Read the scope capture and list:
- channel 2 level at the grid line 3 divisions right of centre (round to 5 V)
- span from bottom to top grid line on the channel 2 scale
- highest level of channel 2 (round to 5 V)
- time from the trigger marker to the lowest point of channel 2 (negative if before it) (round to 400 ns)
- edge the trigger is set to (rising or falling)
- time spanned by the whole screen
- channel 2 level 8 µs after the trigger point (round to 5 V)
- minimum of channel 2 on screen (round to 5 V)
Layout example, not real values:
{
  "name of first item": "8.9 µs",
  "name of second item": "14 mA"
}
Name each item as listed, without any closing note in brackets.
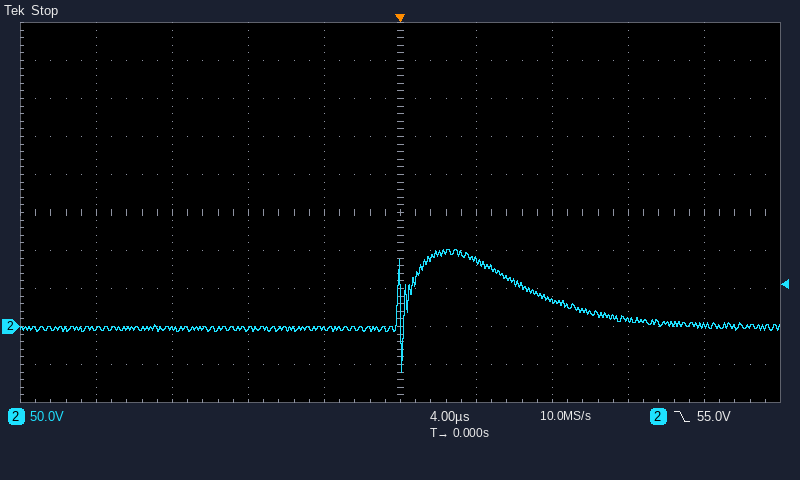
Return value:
{
  "channel 2 level at the grid line 3 divisions right of centre": "10 V",
  "span from bottom to top grid line on the channel 2 scale": "500 V",
  "highest level of channel 2": "100 V",
  "time from the trigger marker to the lowest point of channel 2 (negative if before it)": "0.0 µs",
  "edge the trigger is set to": "falling",
  "time spanned by the whole screen": "40 µs",
  "channel 2 level 8 µs after the trigger point": "35 V",
  "minimum of channel 2 on screen": "-60 V"
}
